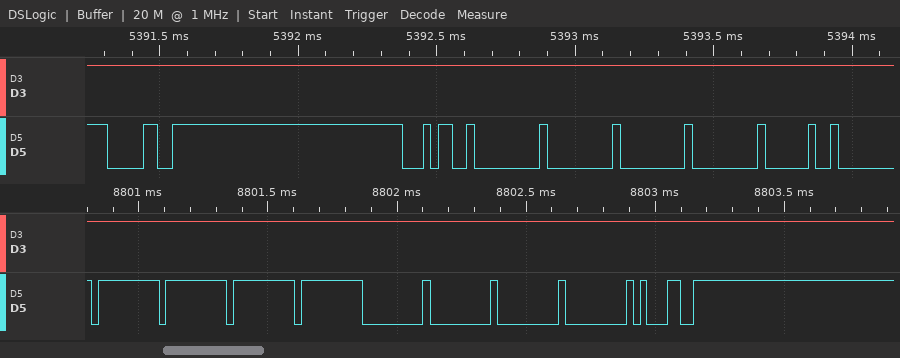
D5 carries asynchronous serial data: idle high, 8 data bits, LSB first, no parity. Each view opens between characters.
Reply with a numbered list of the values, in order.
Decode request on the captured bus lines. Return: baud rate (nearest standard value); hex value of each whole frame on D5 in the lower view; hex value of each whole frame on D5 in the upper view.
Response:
1. 38400 baud
2. FF, FF, FF, FF, 00, 00, 00, 00, 31
3. 30, 34, 00, 00, 00, 00, 20
